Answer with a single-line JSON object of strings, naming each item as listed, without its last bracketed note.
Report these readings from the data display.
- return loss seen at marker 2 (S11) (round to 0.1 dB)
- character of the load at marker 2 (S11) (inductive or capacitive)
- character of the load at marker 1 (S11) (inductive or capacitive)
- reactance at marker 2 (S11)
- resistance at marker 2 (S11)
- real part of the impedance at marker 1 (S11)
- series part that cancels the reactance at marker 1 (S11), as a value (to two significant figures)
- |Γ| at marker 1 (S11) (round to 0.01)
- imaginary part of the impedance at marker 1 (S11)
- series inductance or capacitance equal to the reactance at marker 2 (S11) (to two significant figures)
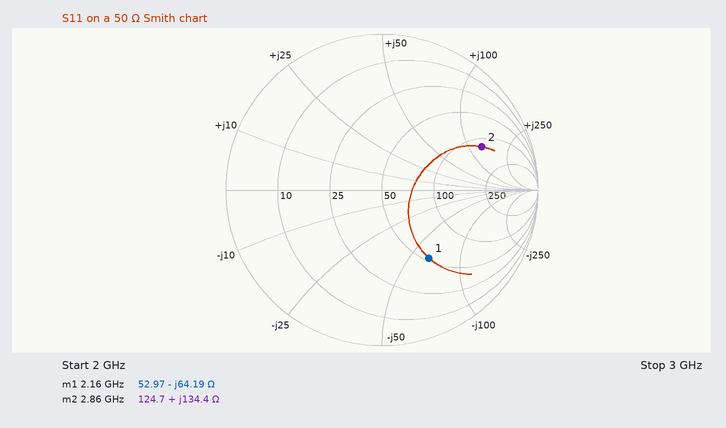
{"return loss seen at marker 2 (S11)": "3.1 dB", "character of the load at marker 2 (S11)": "inductive", "character of the load at marker 1 (S11)": "capacitive", "reactance at marker 2": "+134.4 Ω", "resistance at marker 2": "124.7 Ω", "real part of the impedance at marker 1": "52.97 Ω", "series part that cancels the reactance at marker 1 (S11), as a value": "4.7 nH", "|Γ| at marker 1 (S11)": "0.53", "imaginary part of the impedance at marker 1": "-64.19 Ω", "series inductance or capacitance equal to the reactance at marker 2 (S11)": "7.5 nH"}
